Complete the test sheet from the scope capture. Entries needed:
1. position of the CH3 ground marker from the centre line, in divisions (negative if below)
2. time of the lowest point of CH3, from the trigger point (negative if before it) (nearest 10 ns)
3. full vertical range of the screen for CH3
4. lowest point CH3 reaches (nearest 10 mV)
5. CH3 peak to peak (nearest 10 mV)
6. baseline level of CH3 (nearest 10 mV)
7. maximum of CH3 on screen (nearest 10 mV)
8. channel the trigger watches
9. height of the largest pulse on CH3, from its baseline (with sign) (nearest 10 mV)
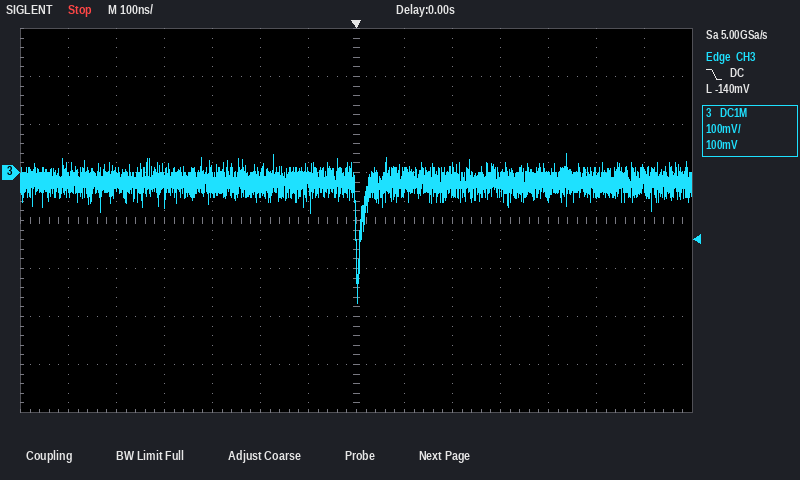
+1.0 div
0 ns
800 mV
-270 mV
310 mV
-20 mV
40 mV
CH3
-250 mV
